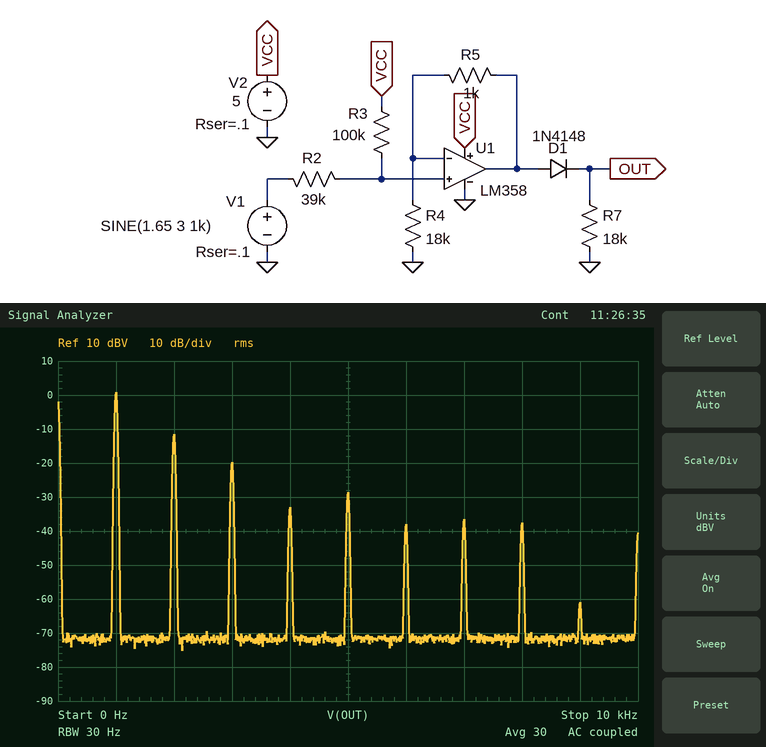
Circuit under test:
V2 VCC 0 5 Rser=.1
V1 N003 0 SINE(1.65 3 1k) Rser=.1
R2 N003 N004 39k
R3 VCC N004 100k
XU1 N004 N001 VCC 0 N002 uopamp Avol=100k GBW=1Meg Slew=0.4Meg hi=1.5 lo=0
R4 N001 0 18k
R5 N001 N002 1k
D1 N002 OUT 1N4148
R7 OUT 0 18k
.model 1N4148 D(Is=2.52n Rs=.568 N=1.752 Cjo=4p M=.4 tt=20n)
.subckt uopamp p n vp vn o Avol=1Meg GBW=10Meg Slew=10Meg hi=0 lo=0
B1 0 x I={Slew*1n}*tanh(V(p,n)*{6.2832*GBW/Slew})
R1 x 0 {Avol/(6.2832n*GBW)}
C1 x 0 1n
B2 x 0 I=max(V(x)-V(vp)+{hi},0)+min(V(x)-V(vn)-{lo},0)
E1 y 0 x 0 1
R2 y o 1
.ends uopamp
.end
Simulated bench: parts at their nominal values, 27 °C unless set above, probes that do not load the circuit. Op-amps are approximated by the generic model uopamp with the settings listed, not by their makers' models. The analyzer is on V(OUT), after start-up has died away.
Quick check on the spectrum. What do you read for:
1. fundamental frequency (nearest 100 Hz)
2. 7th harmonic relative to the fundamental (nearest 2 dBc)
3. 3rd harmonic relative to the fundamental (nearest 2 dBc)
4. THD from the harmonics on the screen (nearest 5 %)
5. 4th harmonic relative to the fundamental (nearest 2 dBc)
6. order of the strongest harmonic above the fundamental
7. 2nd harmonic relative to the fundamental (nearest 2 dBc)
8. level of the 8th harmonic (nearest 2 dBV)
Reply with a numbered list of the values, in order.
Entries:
1. 1.0 kHz
2. -38 dBc
3. -20 dBc
4. 25 %
5. -34 dBc
6. 2
7. -12 dBc
8. -38 dBV
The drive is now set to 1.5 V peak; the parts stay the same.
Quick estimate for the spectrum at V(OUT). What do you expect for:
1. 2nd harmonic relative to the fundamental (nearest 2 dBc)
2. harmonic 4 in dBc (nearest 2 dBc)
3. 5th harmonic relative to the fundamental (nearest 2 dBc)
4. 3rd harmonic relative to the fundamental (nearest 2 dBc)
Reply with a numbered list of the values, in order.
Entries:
1. -20 dBc
2. -30 dBc
3. -42 dBc
4. -24 dBc
